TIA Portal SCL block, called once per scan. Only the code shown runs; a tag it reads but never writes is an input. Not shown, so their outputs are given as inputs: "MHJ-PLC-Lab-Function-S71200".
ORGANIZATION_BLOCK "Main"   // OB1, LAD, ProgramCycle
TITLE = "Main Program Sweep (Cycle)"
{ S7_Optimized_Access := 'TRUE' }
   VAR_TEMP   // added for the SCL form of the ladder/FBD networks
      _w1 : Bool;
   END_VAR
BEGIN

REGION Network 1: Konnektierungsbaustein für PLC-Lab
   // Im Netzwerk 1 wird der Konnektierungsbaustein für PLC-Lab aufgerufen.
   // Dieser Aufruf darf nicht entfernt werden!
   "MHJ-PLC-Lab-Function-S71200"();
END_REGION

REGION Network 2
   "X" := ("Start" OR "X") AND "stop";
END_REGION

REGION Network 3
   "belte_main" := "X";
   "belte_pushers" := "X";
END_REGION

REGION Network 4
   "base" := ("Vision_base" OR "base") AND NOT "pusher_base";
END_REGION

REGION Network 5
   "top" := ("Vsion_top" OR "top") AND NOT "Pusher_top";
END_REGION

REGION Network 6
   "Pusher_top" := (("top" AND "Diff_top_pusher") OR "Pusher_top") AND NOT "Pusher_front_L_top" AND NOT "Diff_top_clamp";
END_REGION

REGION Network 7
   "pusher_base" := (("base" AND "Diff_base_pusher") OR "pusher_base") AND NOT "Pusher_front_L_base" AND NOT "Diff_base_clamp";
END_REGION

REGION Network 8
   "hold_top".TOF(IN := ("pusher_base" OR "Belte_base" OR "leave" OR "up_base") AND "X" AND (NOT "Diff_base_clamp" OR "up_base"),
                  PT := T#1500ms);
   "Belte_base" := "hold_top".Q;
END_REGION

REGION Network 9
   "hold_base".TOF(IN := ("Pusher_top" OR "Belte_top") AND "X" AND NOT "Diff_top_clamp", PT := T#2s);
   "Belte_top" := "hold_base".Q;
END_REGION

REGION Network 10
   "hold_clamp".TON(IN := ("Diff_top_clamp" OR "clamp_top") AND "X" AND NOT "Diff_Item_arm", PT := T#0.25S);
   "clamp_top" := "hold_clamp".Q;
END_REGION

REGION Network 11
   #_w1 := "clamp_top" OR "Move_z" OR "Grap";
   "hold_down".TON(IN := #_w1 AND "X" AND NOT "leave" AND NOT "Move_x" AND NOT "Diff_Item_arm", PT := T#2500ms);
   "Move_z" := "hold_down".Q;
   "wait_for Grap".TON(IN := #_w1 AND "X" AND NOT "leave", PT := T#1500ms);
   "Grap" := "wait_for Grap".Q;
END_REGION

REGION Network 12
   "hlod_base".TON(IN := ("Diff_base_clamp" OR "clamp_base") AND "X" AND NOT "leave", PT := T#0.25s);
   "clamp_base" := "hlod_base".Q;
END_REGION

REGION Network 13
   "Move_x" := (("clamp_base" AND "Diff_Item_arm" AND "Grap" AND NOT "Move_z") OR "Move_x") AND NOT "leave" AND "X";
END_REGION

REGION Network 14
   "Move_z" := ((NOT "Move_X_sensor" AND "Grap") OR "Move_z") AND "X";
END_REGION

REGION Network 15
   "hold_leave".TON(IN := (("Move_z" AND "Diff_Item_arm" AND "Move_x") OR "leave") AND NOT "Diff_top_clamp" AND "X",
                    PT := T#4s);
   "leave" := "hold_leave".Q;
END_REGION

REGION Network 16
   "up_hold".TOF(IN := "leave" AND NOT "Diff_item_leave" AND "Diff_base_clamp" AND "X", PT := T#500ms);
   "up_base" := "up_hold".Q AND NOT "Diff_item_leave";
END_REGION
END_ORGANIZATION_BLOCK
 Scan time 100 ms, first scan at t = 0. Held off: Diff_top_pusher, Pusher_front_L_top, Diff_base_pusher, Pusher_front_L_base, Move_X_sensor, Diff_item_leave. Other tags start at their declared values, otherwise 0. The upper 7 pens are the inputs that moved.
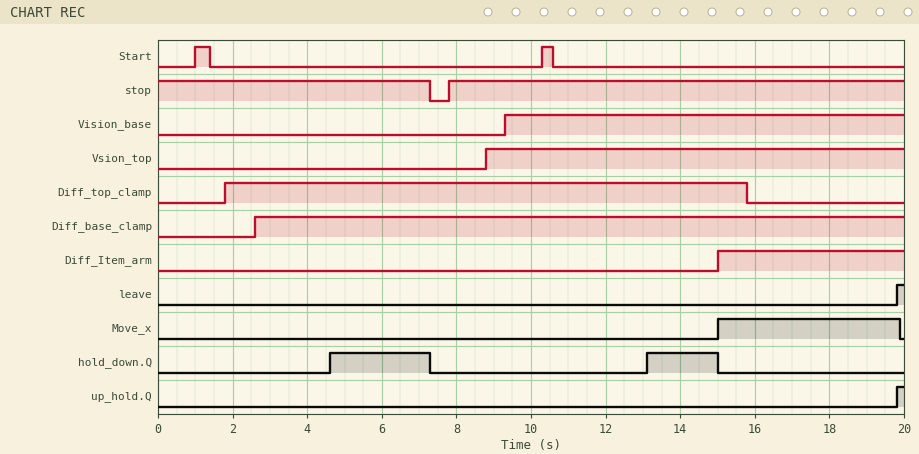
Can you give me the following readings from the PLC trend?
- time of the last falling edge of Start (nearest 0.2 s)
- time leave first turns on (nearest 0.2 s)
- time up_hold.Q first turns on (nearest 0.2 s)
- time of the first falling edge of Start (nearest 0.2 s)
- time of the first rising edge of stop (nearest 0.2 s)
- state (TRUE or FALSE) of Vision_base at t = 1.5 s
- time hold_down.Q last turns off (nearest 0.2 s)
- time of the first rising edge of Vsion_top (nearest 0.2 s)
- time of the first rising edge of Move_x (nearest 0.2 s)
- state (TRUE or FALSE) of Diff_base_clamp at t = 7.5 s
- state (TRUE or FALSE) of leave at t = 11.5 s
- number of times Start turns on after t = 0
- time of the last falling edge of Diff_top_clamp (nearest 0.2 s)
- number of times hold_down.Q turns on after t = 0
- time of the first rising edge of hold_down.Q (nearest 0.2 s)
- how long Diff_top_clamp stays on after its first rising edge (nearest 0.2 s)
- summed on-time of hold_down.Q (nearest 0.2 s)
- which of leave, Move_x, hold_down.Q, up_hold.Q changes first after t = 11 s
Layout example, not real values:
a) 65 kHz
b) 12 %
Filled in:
a) 10.6 s
b) 19.8 s
c) 19.8 s
d) 1.4 s
e) 7.8 s
f) FALSE
g) 15.0 s
h) 8.8 s
i) 15.0 s
j) TRUE
k) FALSE
l) 2
m) 15.8 s
n) 2
o) 4.6 s
p) 14.0 s
q) 4.6 s
r) hold_down.Q
